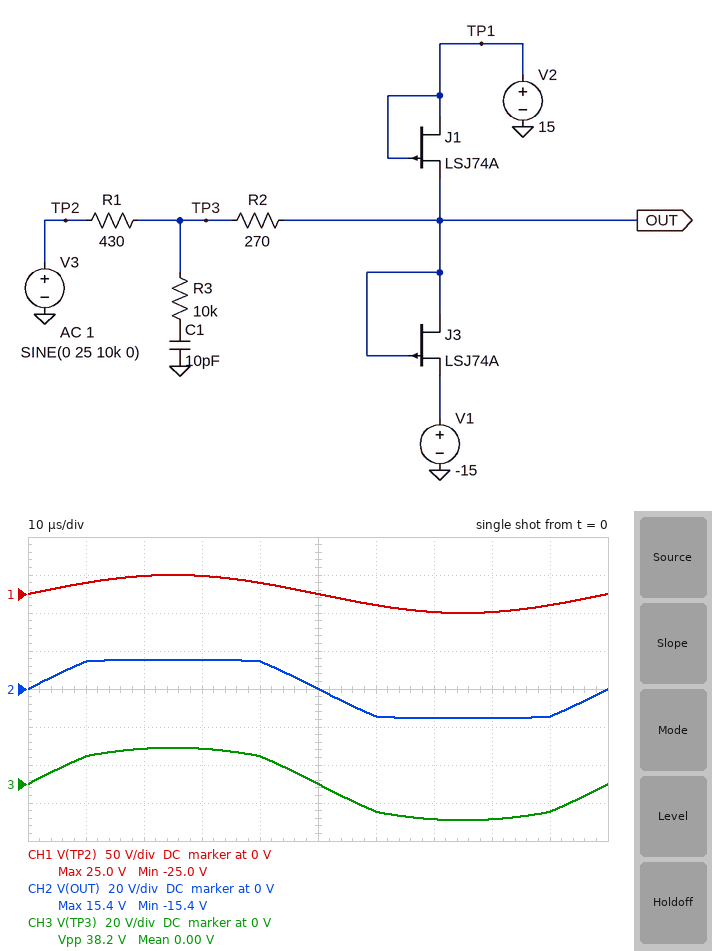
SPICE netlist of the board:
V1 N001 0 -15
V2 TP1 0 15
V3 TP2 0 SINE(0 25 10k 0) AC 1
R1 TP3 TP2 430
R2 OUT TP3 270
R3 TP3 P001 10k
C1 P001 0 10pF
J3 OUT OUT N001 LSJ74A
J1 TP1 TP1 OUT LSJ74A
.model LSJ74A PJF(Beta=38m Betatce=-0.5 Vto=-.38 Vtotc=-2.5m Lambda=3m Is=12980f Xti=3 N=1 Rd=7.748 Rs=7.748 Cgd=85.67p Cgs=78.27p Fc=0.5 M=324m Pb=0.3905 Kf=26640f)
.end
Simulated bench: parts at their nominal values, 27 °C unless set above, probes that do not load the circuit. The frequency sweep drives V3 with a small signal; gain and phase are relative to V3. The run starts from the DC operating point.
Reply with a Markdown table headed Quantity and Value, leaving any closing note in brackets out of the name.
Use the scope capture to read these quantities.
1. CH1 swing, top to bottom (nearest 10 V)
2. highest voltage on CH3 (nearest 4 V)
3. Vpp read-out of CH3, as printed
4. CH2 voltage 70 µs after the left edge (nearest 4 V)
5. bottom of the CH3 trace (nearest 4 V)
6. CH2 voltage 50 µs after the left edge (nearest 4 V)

| Quantity | Value |
|---|---|
| CH1 swing, top to bottom | 50 V |
| highest voltage on CH3 | 20 V |
| Vpp read-out of CH3, as printed | 38.2 V |
| CH2 voltage 70 µs after the left edge | -16 V |
| bottom of the CH3 trace | -20 V |
| CH2 voltage 50 µs after the left edge | 0 V |
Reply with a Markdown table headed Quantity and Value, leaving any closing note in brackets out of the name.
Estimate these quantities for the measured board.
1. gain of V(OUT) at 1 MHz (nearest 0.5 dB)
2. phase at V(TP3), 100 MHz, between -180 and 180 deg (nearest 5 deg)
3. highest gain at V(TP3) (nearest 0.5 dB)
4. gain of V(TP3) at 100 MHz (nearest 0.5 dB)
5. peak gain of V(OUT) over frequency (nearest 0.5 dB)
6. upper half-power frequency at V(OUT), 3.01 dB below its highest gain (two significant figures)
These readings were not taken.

| Quantity | Value |
|---|---|
| gain of V(OUT) at 1 MHz | -0.5 dB |
| phase at V(TP3), 100 MHz, between -180 and 180 deg | -10 deg |
| highest gain at V(TP3) | 0 dB |
| gain of V(TP3) at 100 MHz | -8.0 dB |
| peak gain of V(OUT) over frequency | 0 dB |
| upper half-power frequency at V(OUT), 3.01 dB below its highest gain | 8.6 MHz |
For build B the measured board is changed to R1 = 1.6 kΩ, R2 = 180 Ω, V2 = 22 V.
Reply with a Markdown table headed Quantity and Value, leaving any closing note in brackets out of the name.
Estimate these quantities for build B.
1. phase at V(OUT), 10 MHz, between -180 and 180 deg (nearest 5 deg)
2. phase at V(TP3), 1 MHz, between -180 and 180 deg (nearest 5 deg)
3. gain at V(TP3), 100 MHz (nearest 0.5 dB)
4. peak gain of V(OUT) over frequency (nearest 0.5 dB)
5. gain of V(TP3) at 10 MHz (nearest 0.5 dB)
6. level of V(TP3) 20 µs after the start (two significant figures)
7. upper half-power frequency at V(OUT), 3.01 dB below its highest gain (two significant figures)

| Quantity | Value |
|---|---|
| phase at V(OUT), 10 MHz, between -180 and 180 deg | -65 deg |
| phase at V(TP3), 1 MHz, between -180 and 180 deg | -15 deg |
| gain at V(TP3), 100 MHz | -19.5 dB |
| peak gain of V(OUT) over frequency | -0.5 dB |
| gain of V(TP3) at 10 MHz | -9.0 dB |
| level of V(TP3) 20 µs after the start | 22 V |
| upper half-power frequency at V(OUT), 3.01 dB below its highest gain | 3.2 MHz |
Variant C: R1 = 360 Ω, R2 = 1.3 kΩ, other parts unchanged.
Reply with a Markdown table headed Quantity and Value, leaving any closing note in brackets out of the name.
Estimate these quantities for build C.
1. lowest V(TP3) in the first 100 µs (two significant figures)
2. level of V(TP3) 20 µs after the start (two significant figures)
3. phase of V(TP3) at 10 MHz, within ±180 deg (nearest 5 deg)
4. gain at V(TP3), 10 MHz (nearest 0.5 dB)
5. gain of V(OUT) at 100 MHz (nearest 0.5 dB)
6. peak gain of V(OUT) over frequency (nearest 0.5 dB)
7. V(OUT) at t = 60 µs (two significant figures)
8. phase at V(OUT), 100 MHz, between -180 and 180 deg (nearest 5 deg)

| Quantity | Value |
|---|---|
| lowest V(TP3) in the first 100 µs | -23 V |
| level of V(TP3) 20 µs after the start | 22 V |
| phase of V(TP3) at 10 MHz, within ±180 deg | -5 deg |
| gain at V(TP3), 10 MHz | -2.0 dB |
| gain of V(OUT) at 100 MHz | -28.5 dB |
| peak gain of V(OUT) over frequency | -0.5 dB |
| V(OUT) at t = 60 µs | -14 V |
| phase at V(OUT), 100 MHz, between -180 and 180 deg | -85 deg |
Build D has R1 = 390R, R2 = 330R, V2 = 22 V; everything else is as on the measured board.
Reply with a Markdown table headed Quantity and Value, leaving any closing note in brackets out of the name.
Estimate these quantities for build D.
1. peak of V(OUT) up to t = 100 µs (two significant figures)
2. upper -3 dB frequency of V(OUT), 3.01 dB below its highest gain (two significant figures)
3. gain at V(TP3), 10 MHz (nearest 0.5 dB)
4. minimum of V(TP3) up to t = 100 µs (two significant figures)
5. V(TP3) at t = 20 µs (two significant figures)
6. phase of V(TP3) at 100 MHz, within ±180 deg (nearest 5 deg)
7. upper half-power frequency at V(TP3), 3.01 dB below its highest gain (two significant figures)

| Quantity | Value |
|---|---|
| peak of V(OUT) up to t = 100 µs | 22 V |
| upper -3 dB frequency of V(OUT), 3.01 dB below its highest gain | 9.2 MHz |
| gain at V(TP3), 10 MHz | -2.5 dB |
| minimum of V(TP3) up to t = 100 µs | -20 V |
| V(TP3) at t = 20 µs | 23 V |
| phase of V(TP3) at 100 MHz, within ±180 deg | -5 deg |
| upper half-power frequency at V(TP3), 3.01 dB below its highest gain | 12 MHz |
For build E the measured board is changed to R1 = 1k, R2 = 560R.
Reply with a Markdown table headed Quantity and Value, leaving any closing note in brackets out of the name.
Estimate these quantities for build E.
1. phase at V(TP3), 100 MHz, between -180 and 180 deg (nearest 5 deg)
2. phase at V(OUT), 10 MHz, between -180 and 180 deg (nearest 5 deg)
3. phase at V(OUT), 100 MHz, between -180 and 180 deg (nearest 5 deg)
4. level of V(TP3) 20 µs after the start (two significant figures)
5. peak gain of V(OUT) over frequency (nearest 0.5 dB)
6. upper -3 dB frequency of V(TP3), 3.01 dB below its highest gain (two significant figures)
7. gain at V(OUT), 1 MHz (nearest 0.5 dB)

| Quantity | Value |
|---|---|
| phase at V(TP3), 100 MHz, between -180 and 180 deg | -5 deg |
| phase at V(OUT), 10 MHz, between -180 and 180 deg | -65 deg |
| phase at V(OUT), 100 MHz, between -180 and 180 deg | -85 deg |
| level of V(TP3) 20 µs after the start | 18 V |
| peak gain of V(OUT) over frequency | -0.5 dB |
| upper -3 dB frequency of V(TP3), 3.01 dB below its highest gain | 4.2 MHz |
| gain at V(OUT), 1 MHz | -1.0 dB |
